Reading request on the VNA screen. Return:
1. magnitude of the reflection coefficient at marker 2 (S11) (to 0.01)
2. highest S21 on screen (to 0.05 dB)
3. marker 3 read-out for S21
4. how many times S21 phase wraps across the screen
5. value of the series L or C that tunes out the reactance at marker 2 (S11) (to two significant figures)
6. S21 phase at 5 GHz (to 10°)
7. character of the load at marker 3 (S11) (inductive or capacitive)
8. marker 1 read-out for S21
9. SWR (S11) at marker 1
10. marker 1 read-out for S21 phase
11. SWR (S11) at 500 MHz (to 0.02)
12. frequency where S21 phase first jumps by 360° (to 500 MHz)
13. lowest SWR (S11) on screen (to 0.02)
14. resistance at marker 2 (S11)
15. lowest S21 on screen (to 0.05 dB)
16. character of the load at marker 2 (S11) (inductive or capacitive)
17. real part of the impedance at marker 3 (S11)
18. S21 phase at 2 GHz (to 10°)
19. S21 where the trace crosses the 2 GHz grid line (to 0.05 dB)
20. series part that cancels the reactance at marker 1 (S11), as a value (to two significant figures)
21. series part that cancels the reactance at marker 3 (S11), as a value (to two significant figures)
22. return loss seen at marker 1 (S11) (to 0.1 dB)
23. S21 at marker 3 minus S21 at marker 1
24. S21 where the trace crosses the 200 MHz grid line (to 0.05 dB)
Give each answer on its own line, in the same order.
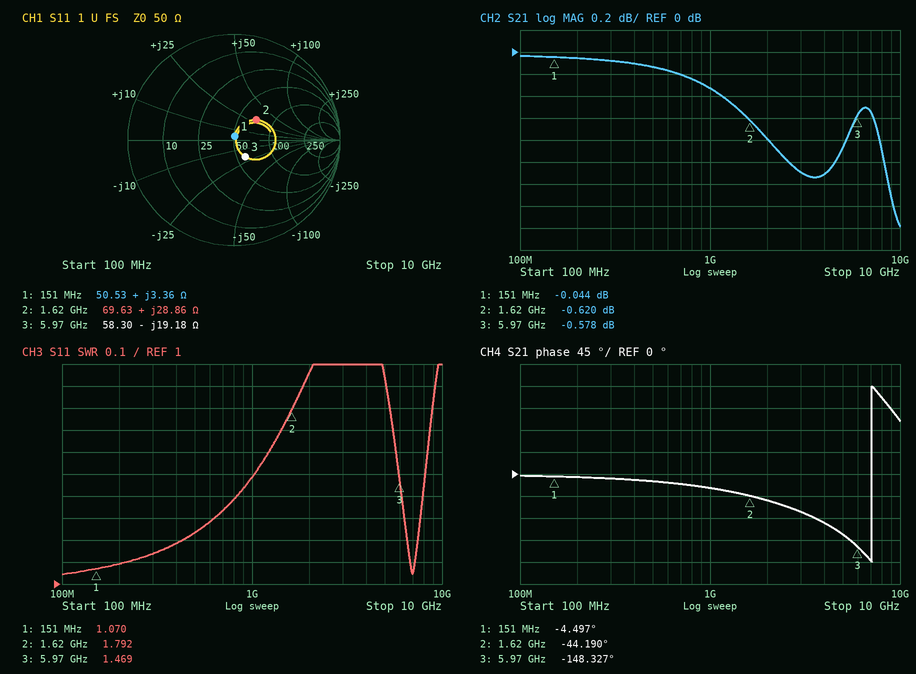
0.28
-0.05 dB
-0.578 dB
1
3.4 pF
-120°
capacitive
-0.044 dB
1.070
-4.497°
1.24
7.0 GHz
1.04
69.63 Ω
-1.60 dB
inductive
58.30 Ω
-50°
-0.80 dB
310 pF
510 pH
29.4 dB
-0.534 dB
-0.05 dB
